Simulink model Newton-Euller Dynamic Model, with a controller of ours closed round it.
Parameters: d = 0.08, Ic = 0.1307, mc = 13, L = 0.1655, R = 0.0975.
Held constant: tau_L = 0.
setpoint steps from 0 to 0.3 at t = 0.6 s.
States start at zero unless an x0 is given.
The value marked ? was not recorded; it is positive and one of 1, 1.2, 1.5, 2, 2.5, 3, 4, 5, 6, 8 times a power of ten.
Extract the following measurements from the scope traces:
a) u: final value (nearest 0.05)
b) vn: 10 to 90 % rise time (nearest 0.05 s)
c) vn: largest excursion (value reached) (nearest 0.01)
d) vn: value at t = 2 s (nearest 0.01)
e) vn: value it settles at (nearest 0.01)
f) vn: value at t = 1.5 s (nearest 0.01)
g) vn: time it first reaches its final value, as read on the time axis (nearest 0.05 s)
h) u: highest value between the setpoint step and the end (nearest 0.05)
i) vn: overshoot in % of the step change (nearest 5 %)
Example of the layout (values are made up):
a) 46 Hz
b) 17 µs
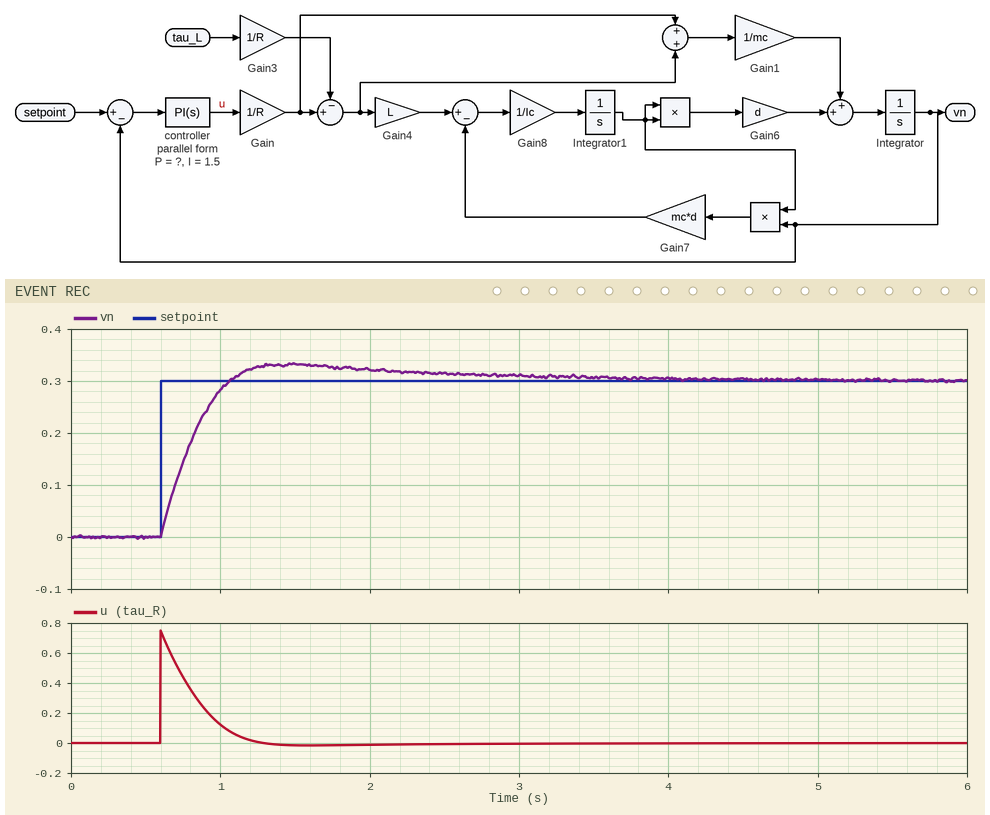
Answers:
a) 0.00
b) 0.35 s
c) 0.33
d) 0.32
e) 0.30
f) 0.33
g) 1.05 s
h) 0.75
i) 10 %
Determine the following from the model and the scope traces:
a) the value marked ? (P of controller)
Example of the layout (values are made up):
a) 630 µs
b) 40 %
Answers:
a) 2.5
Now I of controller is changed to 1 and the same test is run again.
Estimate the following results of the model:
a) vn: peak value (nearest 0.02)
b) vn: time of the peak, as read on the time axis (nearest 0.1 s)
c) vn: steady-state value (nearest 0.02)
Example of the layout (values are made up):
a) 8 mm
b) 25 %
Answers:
a) 0.32
b) 1.5 s
c) 0.30
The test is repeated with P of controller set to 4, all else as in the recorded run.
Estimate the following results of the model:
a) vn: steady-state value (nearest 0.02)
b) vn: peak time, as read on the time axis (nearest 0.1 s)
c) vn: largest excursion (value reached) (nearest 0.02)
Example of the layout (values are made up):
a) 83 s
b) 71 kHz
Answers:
a) 0.30
b) 1.2 s
c) 0.32
